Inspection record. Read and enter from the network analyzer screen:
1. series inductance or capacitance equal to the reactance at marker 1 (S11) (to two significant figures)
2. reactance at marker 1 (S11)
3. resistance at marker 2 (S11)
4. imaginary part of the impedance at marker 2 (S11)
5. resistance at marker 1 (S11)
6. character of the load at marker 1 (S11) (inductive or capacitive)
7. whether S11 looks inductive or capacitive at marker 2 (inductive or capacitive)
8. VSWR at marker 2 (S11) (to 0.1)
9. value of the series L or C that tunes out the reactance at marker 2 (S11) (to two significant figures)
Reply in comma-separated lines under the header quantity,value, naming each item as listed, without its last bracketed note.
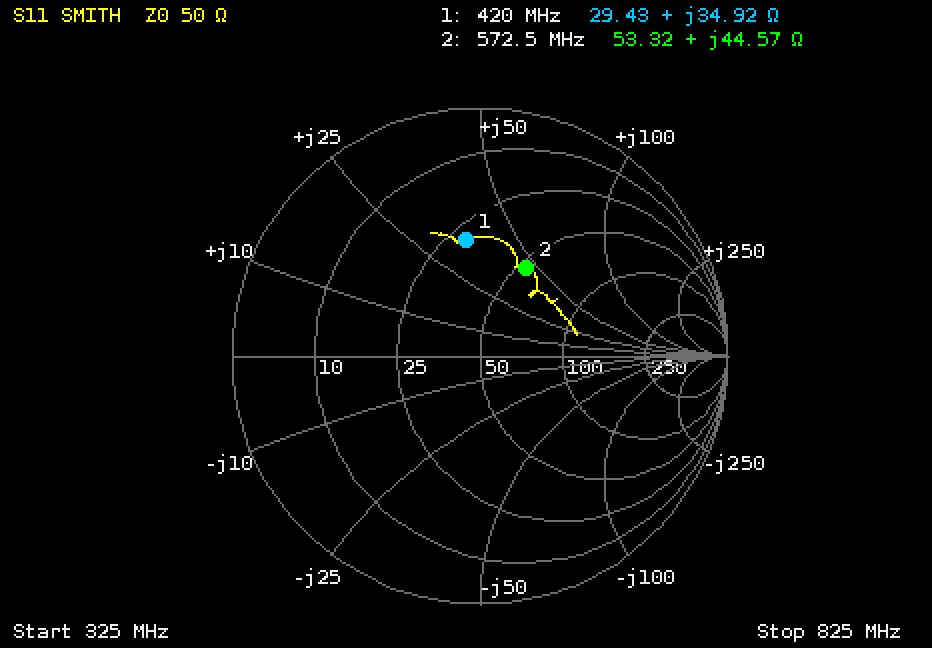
quantity,value
series inductance or capacitance equal to the reactance at marker 1 (S11),13 nH
reactance at marker 1,+34.92 Ω
resistance at marker 2,53.32 Ω
imaginary part of the impedance at marker 2,+44.57 Ω
resistance at marker 1,29.43 Ω
character of the load at marker 1 (S11),inductive
whether S11 looks inductive or capacitive at marker 2,inductive
VSWR at marker 2 (S11),2.3
value of the series L or C that tunes out the reactance at marker 2 (S11),6.2 pF
